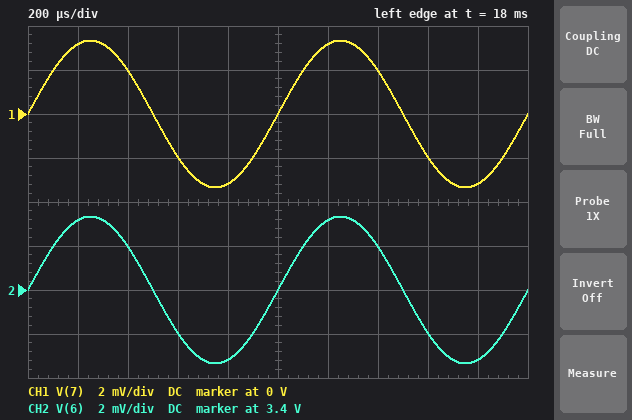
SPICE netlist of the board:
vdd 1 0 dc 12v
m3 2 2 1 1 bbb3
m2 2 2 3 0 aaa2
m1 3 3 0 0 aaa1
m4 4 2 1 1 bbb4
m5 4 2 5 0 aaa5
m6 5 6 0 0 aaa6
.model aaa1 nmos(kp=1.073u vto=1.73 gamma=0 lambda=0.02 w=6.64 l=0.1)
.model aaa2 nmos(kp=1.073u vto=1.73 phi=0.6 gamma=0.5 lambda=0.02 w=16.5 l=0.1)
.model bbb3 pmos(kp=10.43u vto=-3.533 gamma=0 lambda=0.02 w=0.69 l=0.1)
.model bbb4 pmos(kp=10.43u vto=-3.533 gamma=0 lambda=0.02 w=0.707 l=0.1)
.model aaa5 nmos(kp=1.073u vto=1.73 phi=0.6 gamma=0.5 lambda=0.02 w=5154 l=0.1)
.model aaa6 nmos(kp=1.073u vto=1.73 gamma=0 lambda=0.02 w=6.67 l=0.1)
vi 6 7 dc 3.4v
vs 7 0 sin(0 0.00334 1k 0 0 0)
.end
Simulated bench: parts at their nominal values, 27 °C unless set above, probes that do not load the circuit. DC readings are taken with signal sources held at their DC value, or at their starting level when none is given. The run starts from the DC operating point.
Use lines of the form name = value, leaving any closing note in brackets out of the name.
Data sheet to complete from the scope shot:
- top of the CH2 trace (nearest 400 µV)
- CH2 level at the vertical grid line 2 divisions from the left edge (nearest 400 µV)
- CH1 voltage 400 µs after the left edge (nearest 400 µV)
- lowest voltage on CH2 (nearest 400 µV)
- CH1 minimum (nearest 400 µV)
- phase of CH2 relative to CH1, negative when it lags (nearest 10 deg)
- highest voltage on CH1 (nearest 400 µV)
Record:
top of the CH2 trace = 3.4032 V
CH2 level at the vertical grid line 2 divisions from the left edge = 3.4020 V
CH1 voltage 400 µs after the left edge = 2.0 mV
lowest voltage on CH2 = 3.3968 V
CH1 minimum = -3.2 mV
phase of CH2 relative to CH1, negative when it lags = 0 deg
highest voltage on CH1 = 3.2 mV
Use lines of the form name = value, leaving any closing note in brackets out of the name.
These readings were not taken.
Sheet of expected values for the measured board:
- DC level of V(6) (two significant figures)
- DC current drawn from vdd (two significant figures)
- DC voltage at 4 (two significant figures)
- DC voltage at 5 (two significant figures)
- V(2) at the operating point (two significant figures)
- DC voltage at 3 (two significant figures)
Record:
DC level of V(6) = 3.4 V
DC current drawn from vdd = 220 µA
DC voltage at 4 = 7.7 V
DC voltage at 5 = 4.3 V
V(2) at the operating point = 6.8 V
DC voltage at 3 = 3.4 V
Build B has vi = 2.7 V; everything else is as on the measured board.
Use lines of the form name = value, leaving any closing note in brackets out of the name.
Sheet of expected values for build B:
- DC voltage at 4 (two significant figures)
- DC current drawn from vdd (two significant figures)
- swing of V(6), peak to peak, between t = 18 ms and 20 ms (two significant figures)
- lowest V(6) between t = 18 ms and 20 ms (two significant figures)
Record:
DC voltage at 4 = 12 V
DC current drawn from vdd = 140 µA
swing of V(6), peak to peak, between t = 18 ms and 20 ms = 6.7 mV
lowest V(6) between t = 18 ms and 20 ms = 2.7 V
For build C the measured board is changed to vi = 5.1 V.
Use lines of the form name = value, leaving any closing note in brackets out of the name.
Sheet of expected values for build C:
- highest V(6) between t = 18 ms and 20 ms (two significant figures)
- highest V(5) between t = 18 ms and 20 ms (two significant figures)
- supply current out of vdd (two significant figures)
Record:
highest V(6) between t = 18 ms and 20 ms = 5.1 V
highest V(5) between t = 18 ms and 20 ms = 550 mV
supply current out of vdd = 230 µA
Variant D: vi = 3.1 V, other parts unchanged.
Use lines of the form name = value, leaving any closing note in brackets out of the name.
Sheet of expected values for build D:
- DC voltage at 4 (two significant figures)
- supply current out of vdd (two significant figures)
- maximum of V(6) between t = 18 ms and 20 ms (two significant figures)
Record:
DC voltage at 4 = 11 V
supply current out of vdd = 180 µA
maximum of V(6) between t = 18 ms and 20 ms = 3.1 V
